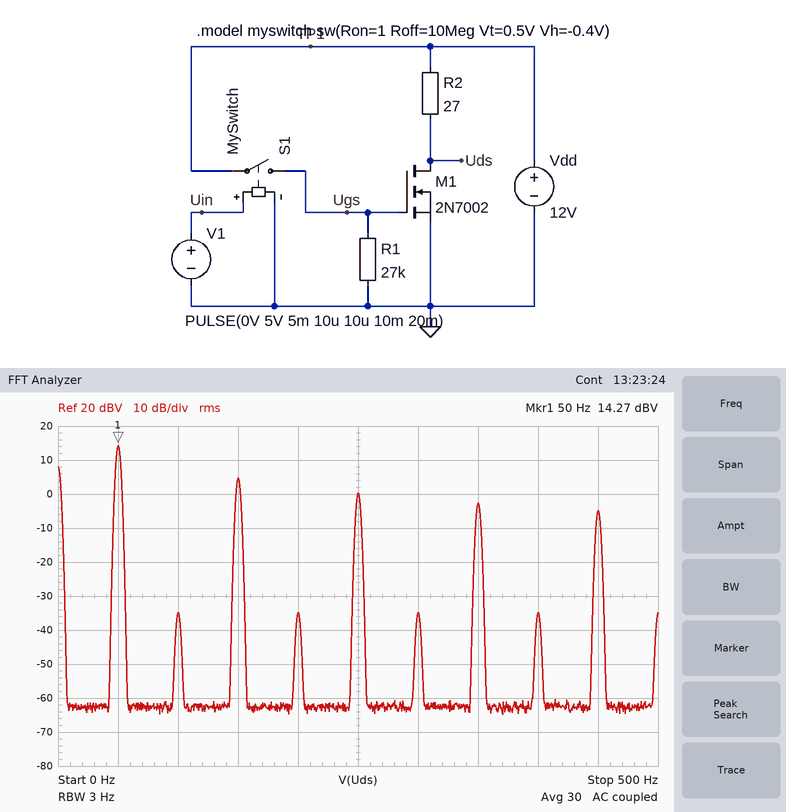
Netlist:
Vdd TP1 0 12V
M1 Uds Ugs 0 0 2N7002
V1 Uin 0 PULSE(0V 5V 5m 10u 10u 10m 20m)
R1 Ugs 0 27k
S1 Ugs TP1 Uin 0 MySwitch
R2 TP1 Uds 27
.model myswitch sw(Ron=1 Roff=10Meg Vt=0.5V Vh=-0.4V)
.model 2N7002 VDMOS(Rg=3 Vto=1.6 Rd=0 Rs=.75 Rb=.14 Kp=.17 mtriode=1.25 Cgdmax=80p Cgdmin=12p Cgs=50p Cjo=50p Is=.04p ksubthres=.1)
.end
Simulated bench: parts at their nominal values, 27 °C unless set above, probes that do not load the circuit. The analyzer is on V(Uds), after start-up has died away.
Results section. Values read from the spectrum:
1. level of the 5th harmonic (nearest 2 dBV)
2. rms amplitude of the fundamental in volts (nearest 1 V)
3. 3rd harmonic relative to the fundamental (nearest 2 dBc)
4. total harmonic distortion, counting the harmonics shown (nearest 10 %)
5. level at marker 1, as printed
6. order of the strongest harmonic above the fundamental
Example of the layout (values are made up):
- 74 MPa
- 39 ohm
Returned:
- 0 dBV
- 5 V
- -10 dBc
- 40 %
- 14.27 dBV
- 3
